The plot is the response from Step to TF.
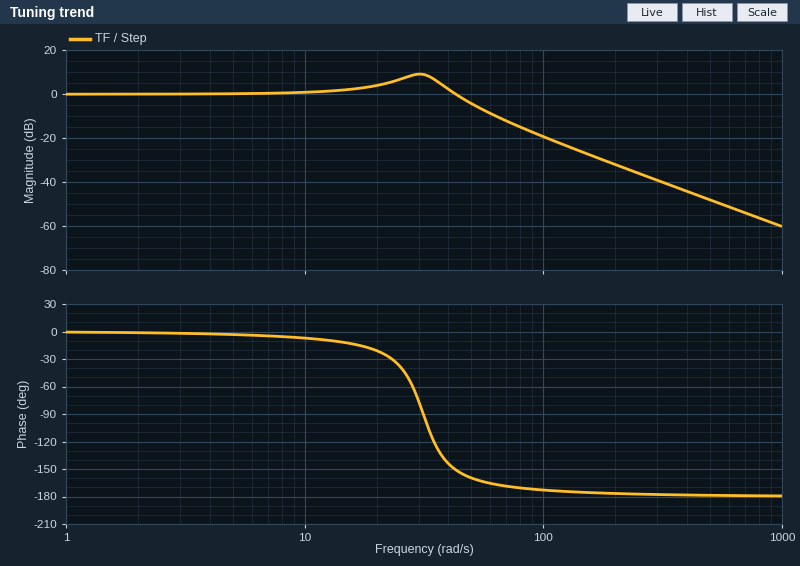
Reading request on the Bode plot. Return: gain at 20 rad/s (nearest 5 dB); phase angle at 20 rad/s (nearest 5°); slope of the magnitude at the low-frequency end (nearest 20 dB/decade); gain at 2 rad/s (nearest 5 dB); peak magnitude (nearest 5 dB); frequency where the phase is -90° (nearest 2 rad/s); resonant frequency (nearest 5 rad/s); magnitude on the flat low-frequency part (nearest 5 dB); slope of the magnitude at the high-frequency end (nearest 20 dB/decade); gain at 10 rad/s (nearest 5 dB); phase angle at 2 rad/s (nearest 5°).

5 dB
-20°
0 dB/decade
0 dB
10 dB
32 rad/s
30 rad/s
0 dB
-40 dB/decade
0 dB
0°
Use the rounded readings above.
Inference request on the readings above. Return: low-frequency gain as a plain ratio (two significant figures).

1.0
